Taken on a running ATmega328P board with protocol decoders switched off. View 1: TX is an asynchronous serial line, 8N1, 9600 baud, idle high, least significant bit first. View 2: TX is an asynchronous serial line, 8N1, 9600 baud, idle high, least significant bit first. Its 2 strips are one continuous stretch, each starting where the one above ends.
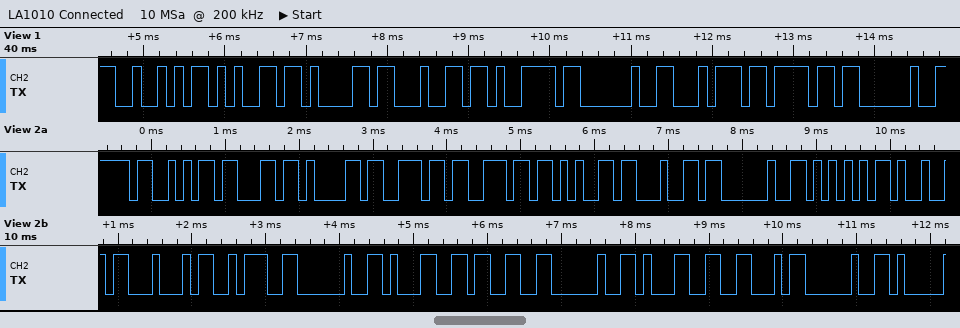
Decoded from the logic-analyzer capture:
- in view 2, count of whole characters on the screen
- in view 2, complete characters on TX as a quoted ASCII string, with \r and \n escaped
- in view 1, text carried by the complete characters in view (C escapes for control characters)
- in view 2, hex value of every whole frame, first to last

19
"Scanned UID: 13 1F "
"Ready to "
53 63 61 6E 6E 65 64 20 55 49 44 3A 20 31 33 20 31 46 20
